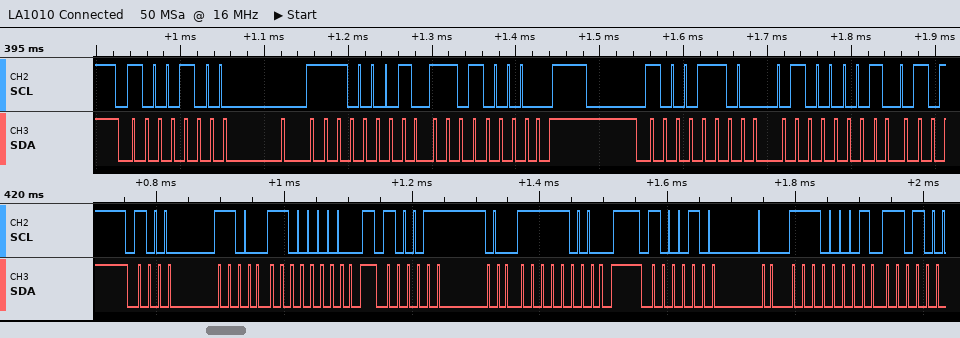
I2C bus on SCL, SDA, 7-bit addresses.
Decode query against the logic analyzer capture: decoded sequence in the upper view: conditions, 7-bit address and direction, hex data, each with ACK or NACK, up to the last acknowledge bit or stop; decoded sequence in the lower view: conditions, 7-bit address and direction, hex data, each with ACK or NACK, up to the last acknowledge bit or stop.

start, address 44 write ACK, E1 ACK, D0 ACK, stop, start, address 46 write ACK, 41 ACK
start, address 46 write ACK, C0 ACK, stop, start, address 46 write ACK, F8 ACK, stop, start, address 44 write ACK, E1 ACK
